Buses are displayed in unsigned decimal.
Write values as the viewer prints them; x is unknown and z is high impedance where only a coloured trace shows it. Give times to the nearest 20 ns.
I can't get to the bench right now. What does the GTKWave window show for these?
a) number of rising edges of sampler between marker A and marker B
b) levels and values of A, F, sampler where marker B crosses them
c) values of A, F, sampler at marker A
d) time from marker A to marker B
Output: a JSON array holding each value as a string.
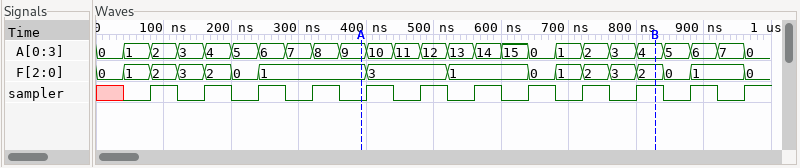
["6", "A=4, F=2, sampler=1", "A=9, F=1, sampler=0", "440 ns"]
